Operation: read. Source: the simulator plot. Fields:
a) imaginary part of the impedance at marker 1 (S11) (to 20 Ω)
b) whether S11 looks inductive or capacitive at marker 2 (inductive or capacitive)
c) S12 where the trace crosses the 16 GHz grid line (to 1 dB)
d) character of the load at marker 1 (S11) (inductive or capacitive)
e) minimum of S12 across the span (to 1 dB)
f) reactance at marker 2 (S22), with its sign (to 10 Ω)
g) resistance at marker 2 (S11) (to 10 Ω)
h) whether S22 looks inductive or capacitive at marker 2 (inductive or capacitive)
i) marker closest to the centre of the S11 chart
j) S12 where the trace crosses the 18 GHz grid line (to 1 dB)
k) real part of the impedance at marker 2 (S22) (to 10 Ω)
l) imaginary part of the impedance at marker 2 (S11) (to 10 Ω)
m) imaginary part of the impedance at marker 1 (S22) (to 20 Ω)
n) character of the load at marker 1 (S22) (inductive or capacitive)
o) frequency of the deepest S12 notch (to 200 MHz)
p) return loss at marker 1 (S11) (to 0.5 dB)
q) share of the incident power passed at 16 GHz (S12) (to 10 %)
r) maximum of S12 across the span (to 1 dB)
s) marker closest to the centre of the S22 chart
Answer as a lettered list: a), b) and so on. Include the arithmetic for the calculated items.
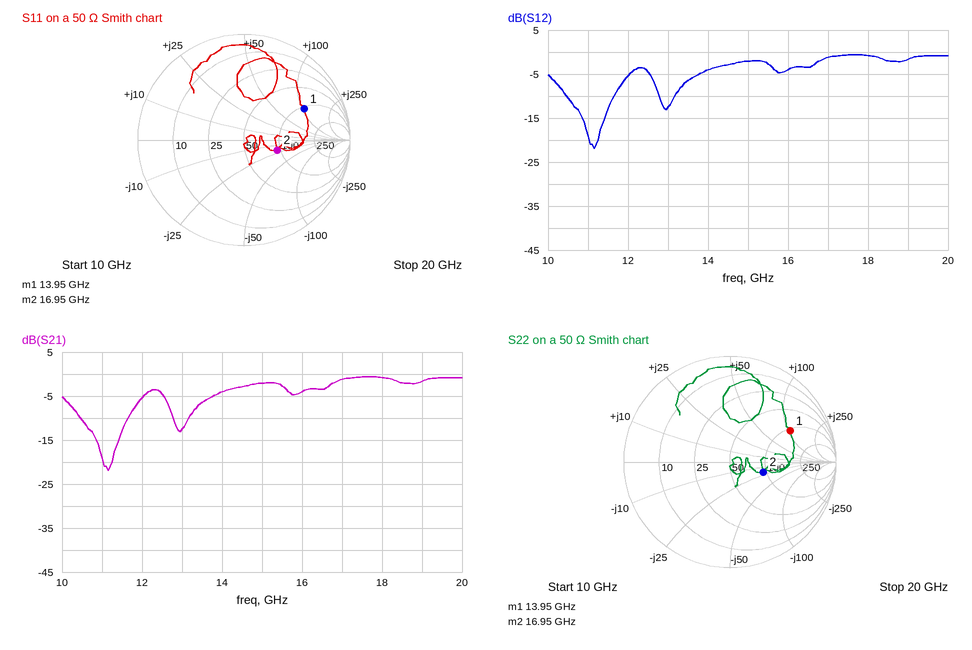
a) +100 Ω
b) capacitive
c) -4 dB
d) inductive
e) -22 dB
f) -20 Ω
g) 90 Ω
h) capacitive
i) marker 2
j) -1 dB
k) 90 Ω
l) -20 Ω
m) +100 Ω
n) inductive
o) 11.2 GHz
p) 4.0 dB
q) 10^(-4/10) ≈ 40 %
r) -1 dB
s) marker 2
